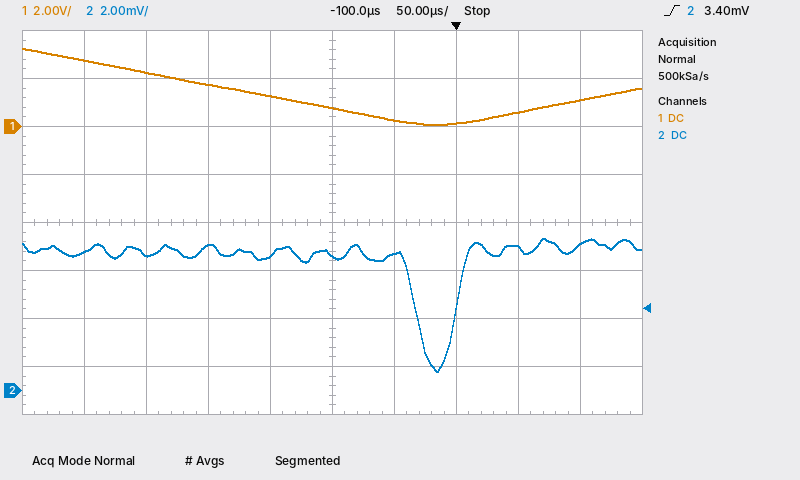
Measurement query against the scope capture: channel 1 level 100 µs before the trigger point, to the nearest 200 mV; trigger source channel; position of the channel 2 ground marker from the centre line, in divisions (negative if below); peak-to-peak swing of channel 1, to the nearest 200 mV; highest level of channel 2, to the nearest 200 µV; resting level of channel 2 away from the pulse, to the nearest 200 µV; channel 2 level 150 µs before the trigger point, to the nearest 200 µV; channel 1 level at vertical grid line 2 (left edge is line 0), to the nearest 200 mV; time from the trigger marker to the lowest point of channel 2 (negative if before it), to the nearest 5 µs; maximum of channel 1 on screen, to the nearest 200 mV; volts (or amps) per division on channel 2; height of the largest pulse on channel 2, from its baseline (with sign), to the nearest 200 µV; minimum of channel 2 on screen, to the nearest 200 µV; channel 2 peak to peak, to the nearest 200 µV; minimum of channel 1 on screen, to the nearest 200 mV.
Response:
800 mV
channel 2
-3.5 div
3.2 V
6.4 mV
5.8 mV
5.6 mV
2.2 V
-15 µs
3.2 V
2 mV
-5.0 mV
800 µV
5.6 mV
0.0 V
